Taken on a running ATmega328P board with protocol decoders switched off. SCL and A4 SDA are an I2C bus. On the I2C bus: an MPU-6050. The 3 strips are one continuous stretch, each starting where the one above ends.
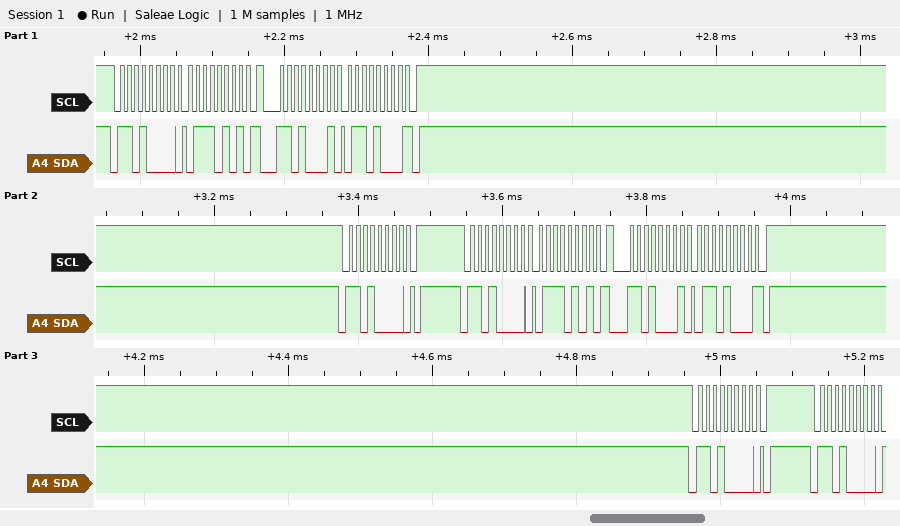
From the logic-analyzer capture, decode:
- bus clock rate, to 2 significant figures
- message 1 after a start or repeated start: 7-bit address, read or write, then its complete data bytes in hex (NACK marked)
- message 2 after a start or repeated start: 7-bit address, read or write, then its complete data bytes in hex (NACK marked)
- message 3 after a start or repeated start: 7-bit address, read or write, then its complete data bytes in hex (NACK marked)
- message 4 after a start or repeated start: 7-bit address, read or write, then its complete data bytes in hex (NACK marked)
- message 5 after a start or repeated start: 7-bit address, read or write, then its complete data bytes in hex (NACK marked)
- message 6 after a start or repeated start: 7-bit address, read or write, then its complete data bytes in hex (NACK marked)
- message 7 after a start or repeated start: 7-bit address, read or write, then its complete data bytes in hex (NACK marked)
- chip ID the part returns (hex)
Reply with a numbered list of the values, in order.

1. 100 kHz
2. 0x68 write: 75
3. 0x68 read: 68 NACK
4. 0x68 write
5. 0x68 write: 75
6. 0x68 read: 68 NACK
7. 0x68 write
8. 0x68 write
9. 0x68
